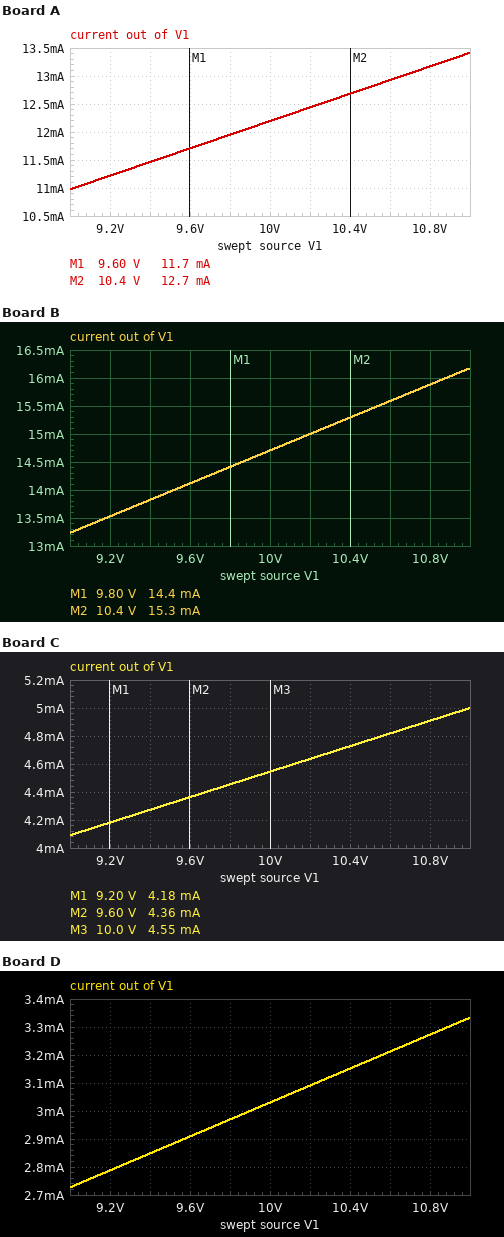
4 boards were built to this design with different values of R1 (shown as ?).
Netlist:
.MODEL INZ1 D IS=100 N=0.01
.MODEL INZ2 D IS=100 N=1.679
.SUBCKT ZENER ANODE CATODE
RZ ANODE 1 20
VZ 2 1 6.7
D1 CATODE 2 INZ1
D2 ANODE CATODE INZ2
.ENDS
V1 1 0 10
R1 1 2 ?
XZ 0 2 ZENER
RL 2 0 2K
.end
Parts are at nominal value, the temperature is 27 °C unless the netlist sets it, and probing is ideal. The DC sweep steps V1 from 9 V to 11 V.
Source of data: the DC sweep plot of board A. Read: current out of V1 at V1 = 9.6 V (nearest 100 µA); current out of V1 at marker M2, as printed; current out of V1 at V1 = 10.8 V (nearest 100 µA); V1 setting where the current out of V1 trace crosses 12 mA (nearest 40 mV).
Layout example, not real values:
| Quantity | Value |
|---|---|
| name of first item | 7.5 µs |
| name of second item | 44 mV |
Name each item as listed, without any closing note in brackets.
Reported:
| Quantity | Value |
|---|---|
| current out of V1 at V1 = 9.6 V | 11.7 mA |
| current out of V1 at marker M2, as printed | 12.7 mA |
| current out of V1 at V1 = 10.8 V | 13.2 mA |
| V1 setting where the current out of V1 trace crosses 12 mA | 9.84 V |
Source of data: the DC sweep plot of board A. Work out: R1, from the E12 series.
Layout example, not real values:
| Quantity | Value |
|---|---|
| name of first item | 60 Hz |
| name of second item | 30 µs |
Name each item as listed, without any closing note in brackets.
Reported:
| Quantity | Value |
|---|---|
| R1, from the E12 series | 820 Ω |
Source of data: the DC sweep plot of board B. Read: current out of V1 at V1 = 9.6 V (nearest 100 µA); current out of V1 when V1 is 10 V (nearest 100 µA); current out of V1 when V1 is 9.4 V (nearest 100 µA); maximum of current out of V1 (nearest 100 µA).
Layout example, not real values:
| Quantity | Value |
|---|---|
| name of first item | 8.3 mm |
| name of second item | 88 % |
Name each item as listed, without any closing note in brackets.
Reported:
| Quantity | Value |
|---|---|
| current out of V1 at V1 = 9.6 V | 14.1 mA |
| current out of V1 when V1 is 10 V | 14.7 mA |
| current out of V1 when V1 is 9.4 V | 13.8 mA |
| maximum of current out of V1 | 16.2 mA |
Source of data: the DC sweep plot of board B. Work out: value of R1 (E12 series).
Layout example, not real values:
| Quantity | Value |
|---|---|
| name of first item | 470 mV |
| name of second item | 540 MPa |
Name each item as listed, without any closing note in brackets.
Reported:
| Quantity | Value |
|---|---|
| value of R1 | 680 Ω |
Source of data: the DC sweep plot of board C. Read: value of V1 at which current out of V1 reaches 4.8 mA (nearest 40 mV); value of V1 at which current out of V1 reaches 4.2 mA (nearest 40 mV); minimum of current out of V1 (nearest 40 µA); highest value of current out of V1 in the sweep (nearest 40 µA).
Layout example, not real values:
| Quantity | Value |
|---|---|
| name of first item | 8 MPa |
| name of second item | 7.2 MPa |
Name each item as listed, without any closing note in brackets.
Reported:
| Quantity | Value |
|---|---|
| value of V1 at which current out of V1 reaches 4.8 mA | 10.56 V |
| value of V1 at which current out of V1 reaches 4.2 mA | 9.24 V |
| minimum of current out of V1 | 4.08 mA |
| highest value of current out of V1 in the sweep | 5.00 mA |
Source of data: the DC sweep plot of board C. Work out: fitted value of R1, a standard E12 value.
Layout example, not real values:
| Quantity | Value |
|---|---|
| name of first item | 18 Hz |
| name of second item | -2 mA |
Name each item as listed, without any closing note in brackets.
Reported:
| Quantity | Value |
|---|---|
| fitted value of R1, a standard E12 value | 2.2 kΩ |
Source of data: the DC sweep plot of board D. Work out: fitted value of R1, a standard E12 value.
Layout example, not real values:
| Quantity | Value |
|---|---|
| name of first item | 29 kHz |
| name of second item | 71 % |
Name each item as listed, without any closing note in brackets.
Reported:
| Quantity | Value |
|---|---|
| fitted value of R1, a standard E12 value | 3.3 kΩ |
